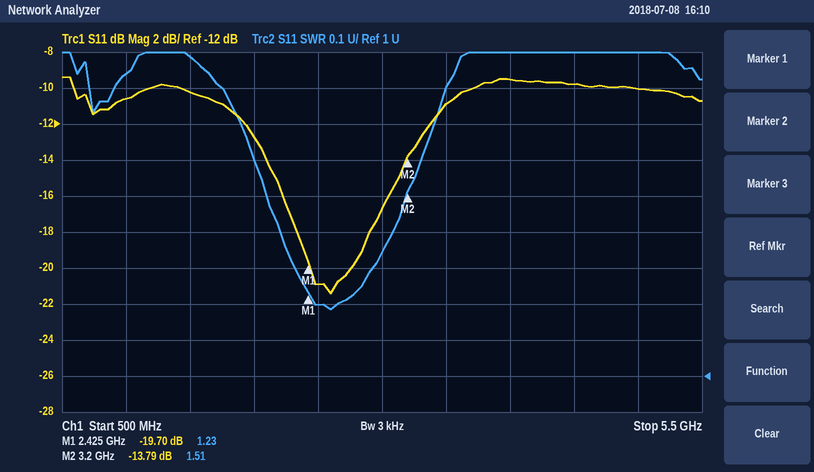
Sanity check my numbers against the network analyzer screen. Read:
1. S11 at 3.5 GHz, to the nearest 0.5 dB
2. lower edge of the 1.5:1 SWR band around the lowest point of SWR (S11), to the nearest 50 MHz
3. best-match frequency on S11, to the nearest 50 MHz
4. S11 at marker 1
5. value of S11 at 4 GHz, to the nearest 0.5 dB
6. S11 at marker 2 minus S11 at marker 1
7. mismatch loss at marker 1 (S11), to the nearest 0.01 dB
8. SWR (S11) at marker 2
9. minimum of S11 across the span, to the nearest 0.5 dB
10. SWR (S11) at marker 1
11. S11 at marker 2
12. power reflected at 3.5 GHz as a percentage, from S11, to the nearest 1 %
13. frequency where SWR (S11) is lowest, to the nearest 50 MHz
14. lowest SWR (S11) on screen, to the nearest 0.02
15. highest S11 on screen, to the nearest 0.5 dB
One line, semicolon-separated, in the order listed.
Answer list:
-11.0 dB; 2.10 GHz; 2.60 GHz; -19.70 dB; -9.5 dB; 5.91 dB; 0.05 dB; 1.51; -21.5 dB; 1.23; -13.79 dB; 8 %; 2.60 GHz; 1.18; -9.5 dB
